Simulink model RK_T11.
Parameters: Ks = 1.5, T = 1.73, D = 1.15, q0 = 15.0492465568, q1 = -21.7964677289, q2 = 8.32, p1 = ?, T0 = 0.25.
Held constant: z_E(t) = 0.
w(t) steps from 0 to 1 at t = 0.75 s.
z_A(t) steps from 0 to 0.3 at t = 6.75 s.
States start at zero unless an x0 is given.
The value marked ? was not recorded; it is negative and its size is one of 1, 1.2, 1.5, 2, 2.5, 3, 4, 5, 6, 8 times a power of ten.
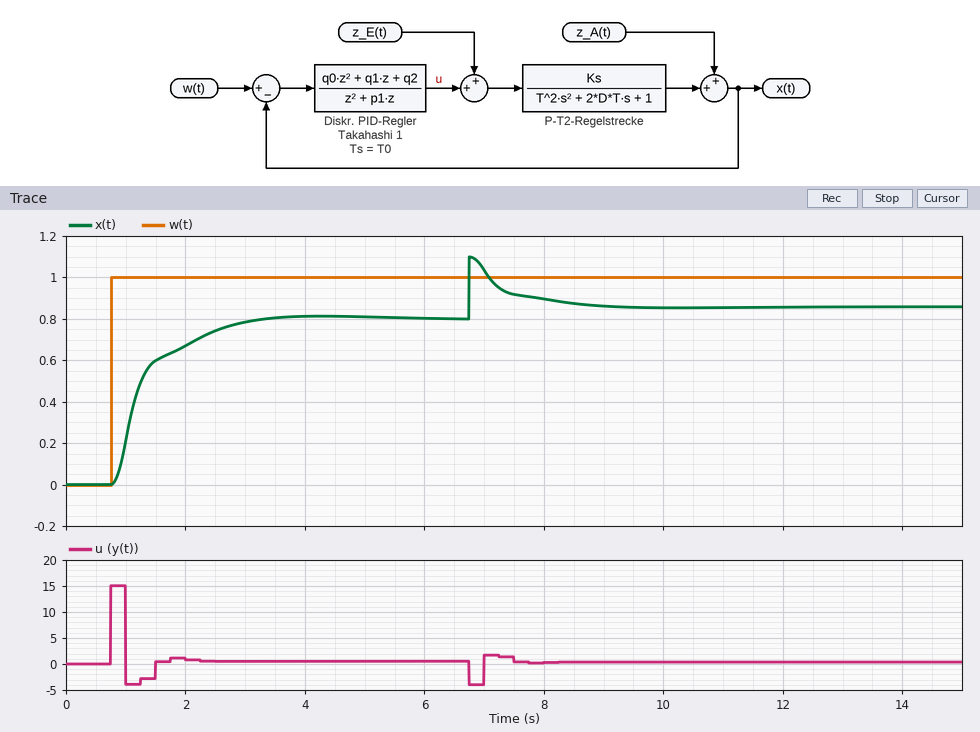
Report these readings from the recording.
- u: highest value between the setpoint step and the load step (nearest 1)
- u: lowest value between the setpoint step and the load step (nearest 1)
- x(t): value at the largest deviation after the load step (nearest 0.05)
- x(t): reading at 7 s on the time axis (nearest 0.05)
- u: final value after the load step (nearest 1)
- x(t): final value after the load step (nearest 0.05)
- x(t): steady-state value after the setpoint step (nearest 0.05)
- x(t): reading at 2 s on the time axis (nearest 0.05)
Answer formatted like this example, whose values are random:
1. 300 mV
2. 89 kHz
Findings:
1. 15
2. -4
3. 1.10
4. 1.05
5. 0
6. 0.85
7. 0.80
8. 0.65
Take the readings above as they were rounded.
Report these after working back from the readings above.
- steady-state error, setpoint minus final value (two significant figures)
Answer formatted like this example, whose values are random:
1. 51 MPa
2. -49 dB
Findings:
1. 0.20
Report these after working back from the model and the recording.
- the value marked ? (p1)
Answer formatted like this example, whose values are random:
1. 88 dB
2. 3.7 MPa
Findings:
1. -0.4
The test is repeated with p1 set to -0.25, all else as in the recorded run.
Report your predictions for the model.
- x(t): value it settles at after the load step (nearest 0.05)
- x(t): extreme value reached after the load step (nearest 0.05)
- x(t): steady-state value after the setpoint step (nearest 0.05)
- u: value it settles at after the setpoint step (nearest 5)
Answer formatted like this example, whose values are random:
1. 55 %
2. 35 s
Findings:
1. 0.85
2. 1.05
3. 0.75
4. 0
